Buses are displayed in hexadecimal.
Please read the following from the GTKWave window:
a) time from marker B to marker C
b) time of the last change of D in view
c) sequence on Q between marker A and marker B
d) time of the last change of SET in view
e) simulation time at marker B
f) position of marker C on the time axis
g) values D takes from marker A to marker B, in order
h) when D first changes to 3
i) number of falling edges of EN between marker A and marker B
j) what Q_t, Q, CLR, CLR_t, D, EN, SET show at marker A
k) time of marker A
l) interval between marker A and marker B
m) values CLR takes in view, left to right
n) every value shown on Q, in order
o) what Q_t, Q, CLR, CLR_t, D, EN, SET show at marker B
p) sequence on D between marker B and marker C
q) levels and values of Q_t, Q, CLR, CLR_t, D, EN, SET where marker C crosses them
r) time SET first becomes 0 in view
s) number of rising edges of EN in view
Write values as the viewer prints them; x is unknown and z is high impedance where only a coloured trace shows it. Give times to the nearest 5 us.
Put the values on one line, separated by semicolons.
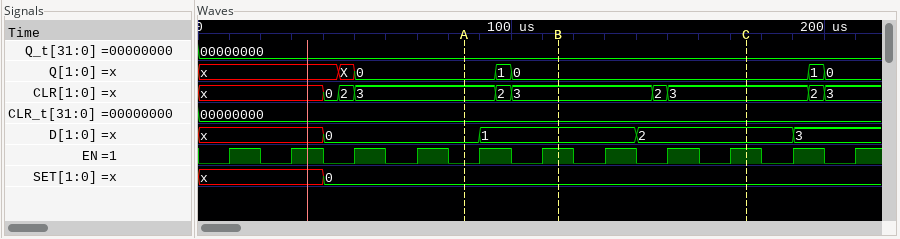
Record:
60 us; 190 us; 0, 1, 0; 40 us; 115 us; 175 us; 0, 1; 190 us; 1; Q_t=00000000, Q=0, CLR=3, CLR_t=00000000, D=0, EN=0, SET=0; 85 us; 30 us; x, 0, 2, 3, 2, 3, 2, 3, 2, 3; x, X, 0, 1, 0, 1, 0; Q_t=00000000, Q=0, CLR=3, CLR_t=00000000, D=1, EN=1, SET=0; 1, 2; Q_t=00000000, Q=0, CLR=3, CLR_t=00000000, D=2, EN=1, SET=0; 40 us; 11
